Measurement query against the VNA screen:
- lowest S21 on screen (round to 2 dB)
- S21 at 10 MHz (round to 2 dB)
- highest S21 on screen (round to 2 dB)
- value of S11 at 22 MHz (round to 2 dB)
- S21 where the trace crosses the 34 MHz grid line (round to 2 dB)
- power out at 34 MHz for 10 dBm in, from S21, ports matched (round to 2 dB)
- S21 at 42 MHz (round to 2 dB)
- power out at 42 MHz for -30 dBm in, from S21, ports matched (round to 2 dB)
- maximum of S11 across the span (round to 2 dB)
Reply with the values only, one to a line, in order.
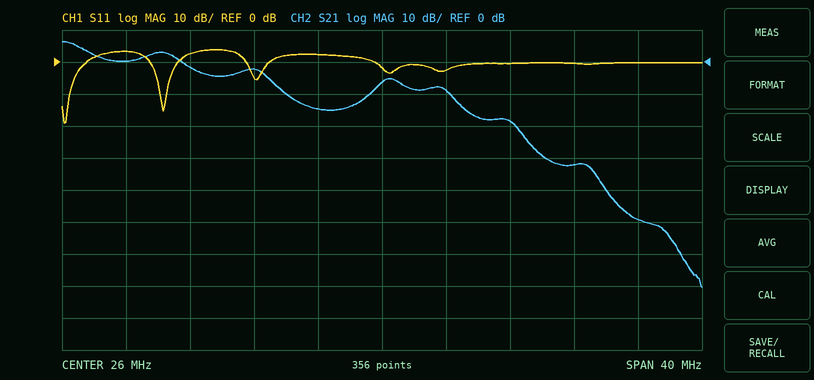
-70 dB
0 dB
6 dB
2 dB
-18 dB
-8 dBm
-50 dB
-80 dBm
4 dB
